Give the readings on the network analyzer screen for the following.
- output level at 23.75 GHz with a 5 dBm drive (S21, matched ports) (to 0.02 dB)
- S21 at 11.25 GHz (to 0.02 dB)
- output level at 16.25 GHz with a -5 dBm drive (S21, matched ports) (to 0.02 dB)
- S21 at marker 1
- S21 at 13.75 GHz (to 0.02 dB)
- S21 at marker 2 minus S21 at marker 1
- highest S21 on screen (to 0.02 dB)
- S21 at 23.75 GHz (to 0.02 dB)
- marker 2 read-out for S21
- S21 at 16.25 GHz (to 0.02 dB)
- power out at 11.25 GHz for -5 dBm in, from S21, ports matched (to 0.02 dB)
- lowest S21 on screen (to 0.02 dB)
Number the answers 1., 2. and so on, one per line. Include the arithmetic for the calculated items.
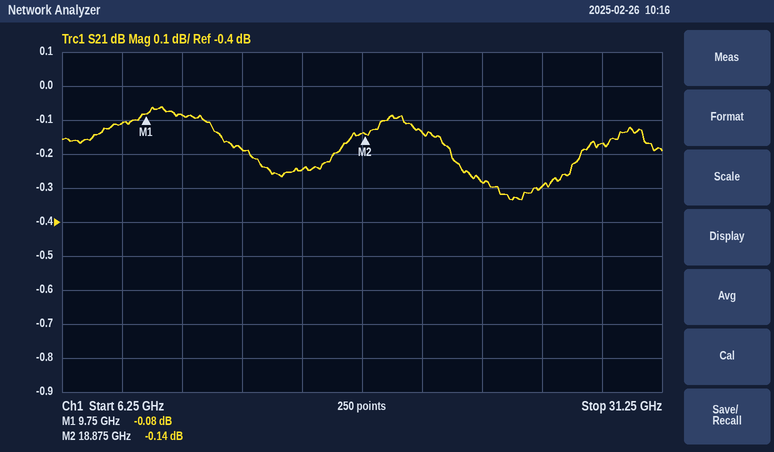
1. 5 dBm + (-0.28 dB) = 4.72 dBm
2. -0.08 dB
3. -5 dBm + (-0.24 dB) = -5.24 dBm
4. -0.08 dB
5. -0.18 dB
6. -0.14 − (-0.08) = -0.06 dB
7. -0.06 dB
8. -0.28 dB
9. -0.14 dB
10. -0.24 dB
11. -5 dBm + (-0.08 dB) = -5.08 dBm
12. -0.34 dB
